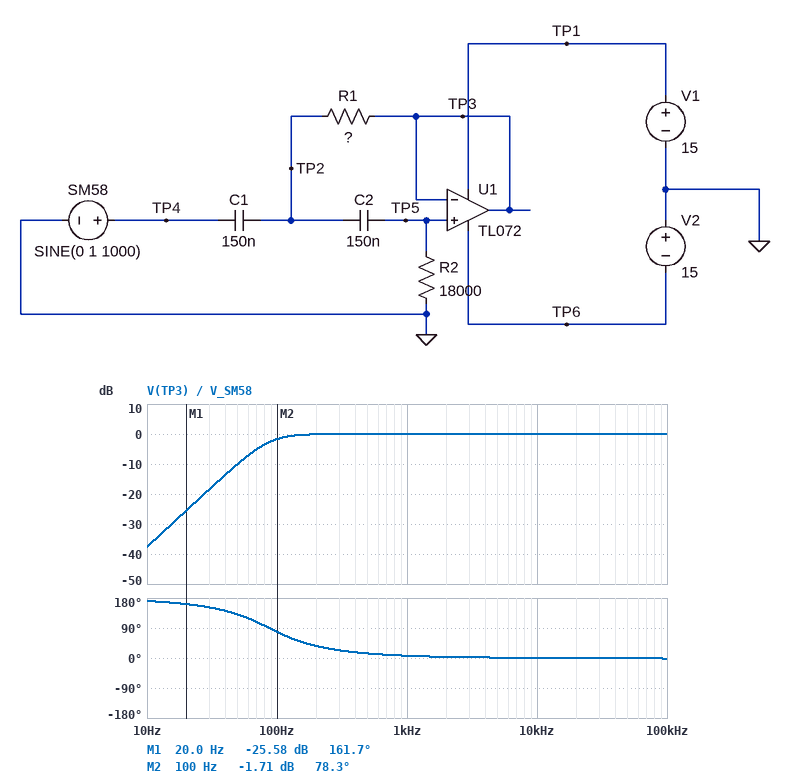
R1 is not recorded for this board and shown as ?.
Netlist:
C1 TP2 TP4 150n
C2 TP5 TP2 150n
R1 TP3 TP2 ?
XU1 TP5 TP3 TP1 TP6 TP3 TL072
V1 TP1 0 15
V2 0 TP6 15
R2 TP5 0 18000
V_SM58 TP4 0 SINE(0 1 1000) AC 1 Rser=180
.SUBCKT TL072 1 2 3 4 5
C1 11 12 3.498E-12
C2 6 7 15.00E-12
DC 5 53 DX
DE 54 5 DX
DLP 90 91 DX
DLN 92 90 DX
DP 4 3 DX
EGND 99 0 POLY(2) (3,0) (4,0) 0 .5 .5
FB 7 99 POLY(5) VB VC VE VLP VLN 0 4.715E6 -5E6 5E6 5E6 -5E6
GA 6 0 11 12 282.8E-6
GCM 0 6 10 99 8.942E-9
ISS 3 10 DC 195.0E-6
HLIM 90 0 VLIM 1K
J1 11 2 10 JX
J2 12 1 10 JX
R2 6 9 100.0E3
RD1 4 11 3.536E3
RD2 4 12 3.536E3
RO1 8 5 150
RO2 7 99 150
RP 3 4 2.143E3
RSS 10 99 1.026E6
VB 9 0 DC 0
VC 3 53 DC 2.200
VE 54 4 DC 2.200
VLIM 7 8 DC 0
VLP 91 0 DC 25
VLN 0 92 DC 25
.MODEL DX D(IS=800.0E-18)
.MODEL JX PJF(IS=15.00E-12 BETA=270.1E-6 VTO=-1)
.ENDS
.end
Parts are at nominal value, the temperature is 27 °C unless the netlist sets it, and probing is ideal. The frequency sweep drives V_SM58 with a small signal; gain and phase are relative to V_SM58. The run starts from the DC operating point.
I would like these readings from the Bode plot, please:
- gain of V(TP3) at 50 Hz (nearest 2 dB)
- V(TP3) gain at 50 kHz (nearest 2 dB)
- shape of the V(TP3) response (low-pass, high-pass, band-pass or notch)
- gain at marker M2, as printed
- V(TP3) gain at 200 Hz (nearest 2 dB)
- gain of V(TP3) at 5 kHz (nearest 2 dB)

-10 dB
0 dB
high-pass
-1.71 dB
0 dB
0 dB
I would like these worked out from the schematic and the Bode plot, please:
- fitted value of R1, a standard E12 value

8.2 kΩ
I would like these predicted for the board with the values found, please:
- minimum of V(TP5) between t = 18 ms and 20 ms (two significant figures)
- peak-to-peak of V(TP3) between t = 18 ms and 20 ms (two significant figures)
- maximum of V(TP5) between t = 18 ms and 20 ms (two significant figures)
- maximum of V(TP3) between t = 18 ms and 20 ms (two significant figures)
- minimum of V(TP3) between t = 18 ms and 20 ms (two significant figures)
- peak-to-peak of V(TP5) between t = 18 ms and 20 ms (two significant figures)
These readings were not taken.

-990 mV
2.0 V
990 mV
990 mV
-990 mV
2.0 V
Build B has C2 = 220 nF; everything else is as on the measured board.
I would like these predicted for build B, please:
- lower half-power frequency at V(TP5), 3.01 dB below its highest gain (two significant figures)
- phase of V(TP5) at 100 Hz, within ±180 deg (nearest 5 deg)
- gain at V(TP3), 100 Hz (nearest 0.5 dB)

70 Hz
65 deg
-1.0 dB
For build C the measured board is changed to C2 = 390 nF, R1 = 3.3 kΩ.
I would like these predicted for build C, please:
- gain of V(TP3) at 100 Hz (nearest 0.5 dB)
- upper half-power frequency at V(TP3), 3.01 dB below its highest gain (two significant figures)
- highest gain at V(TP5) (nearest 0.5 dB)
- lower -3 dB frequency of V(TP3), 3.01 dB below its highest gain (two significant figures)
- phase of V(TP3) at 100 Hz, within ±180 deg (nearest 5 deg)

1.0 dB
3.4 MHz
1.5 dB
72 Hz
70 deg
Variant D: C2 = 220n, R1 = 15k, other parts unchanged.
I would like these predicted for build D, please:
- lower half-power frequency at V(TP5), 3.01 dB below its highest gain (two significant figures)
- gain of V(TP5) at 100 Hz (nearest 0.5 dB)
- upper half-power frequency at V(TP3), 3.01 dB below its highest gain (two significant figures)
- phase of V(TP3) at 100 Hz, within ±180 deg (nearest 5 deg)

74 Hz
-2.0 dB
4.7 MHz
55 deg
